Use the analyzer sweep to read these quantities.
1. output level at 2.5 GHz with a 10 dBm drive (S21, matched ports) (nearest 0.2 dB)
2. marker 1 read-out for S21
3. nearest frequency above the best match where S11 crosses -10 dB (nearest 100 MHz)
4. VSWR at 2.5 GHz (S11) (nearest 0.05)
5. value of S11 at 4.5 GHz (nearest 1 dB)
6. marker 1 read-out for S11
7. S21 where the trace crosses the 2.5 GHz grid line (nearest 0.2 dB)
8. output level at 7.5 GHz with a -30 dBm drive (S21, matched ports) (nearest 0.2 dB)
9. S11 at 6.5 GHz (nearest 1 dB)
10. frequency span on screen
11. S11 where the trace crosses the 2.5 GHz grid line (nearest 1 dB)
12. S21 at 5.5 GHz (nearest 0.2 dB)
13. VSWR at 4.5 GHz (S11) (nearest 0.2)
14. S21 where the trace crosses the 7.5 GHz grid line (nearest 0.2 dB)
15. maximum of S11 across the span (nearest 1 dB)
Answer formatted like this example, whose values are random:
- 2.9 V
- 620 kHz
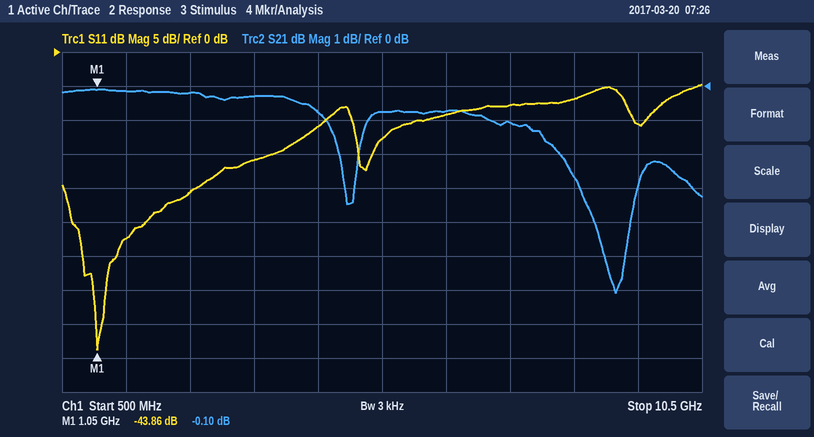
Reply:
- 9.8 dBm
- -0.10 dB
- 4.6 GHz
- 1.20
- -11 dB
- -43.86 dB
- -0.2 dB
- -31.0 dBm
- -9 dB
- 10 GHz
- -21 dB
- -0.8 dB
- 1.8
- -1.0 dB
- -5 dB
